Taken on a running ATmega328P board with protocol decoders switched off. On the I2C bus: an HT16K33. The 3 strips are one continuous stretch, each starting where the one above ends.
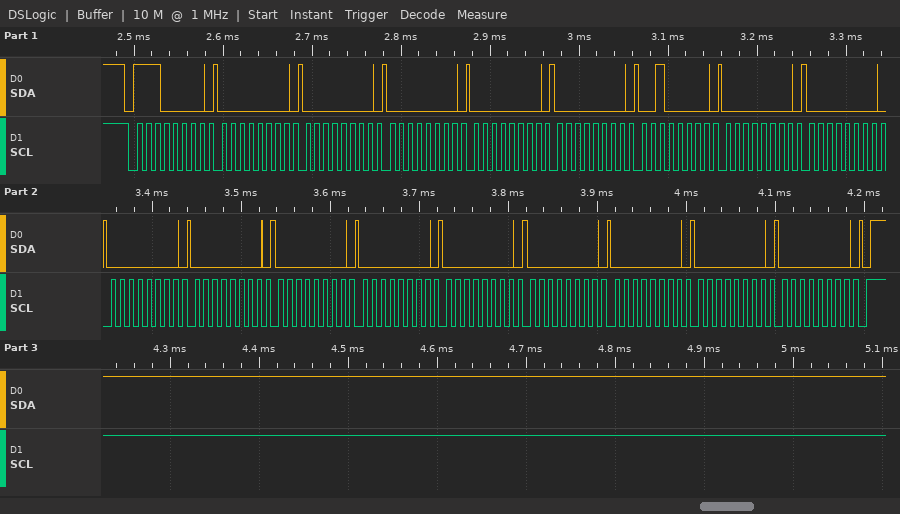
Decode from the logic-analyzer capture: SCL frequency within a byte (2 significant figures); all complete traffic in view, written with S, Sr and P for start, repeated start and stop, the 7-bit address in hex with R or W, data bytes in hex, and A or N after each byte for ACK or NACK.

100 kHz
S 70W A 00 A 00 A 00 A 00 A 00 A 20 A 00 A 00 A 00 A 00 A 00 A 00 A 00 A 00 A 00 A 00 A 00 A P
